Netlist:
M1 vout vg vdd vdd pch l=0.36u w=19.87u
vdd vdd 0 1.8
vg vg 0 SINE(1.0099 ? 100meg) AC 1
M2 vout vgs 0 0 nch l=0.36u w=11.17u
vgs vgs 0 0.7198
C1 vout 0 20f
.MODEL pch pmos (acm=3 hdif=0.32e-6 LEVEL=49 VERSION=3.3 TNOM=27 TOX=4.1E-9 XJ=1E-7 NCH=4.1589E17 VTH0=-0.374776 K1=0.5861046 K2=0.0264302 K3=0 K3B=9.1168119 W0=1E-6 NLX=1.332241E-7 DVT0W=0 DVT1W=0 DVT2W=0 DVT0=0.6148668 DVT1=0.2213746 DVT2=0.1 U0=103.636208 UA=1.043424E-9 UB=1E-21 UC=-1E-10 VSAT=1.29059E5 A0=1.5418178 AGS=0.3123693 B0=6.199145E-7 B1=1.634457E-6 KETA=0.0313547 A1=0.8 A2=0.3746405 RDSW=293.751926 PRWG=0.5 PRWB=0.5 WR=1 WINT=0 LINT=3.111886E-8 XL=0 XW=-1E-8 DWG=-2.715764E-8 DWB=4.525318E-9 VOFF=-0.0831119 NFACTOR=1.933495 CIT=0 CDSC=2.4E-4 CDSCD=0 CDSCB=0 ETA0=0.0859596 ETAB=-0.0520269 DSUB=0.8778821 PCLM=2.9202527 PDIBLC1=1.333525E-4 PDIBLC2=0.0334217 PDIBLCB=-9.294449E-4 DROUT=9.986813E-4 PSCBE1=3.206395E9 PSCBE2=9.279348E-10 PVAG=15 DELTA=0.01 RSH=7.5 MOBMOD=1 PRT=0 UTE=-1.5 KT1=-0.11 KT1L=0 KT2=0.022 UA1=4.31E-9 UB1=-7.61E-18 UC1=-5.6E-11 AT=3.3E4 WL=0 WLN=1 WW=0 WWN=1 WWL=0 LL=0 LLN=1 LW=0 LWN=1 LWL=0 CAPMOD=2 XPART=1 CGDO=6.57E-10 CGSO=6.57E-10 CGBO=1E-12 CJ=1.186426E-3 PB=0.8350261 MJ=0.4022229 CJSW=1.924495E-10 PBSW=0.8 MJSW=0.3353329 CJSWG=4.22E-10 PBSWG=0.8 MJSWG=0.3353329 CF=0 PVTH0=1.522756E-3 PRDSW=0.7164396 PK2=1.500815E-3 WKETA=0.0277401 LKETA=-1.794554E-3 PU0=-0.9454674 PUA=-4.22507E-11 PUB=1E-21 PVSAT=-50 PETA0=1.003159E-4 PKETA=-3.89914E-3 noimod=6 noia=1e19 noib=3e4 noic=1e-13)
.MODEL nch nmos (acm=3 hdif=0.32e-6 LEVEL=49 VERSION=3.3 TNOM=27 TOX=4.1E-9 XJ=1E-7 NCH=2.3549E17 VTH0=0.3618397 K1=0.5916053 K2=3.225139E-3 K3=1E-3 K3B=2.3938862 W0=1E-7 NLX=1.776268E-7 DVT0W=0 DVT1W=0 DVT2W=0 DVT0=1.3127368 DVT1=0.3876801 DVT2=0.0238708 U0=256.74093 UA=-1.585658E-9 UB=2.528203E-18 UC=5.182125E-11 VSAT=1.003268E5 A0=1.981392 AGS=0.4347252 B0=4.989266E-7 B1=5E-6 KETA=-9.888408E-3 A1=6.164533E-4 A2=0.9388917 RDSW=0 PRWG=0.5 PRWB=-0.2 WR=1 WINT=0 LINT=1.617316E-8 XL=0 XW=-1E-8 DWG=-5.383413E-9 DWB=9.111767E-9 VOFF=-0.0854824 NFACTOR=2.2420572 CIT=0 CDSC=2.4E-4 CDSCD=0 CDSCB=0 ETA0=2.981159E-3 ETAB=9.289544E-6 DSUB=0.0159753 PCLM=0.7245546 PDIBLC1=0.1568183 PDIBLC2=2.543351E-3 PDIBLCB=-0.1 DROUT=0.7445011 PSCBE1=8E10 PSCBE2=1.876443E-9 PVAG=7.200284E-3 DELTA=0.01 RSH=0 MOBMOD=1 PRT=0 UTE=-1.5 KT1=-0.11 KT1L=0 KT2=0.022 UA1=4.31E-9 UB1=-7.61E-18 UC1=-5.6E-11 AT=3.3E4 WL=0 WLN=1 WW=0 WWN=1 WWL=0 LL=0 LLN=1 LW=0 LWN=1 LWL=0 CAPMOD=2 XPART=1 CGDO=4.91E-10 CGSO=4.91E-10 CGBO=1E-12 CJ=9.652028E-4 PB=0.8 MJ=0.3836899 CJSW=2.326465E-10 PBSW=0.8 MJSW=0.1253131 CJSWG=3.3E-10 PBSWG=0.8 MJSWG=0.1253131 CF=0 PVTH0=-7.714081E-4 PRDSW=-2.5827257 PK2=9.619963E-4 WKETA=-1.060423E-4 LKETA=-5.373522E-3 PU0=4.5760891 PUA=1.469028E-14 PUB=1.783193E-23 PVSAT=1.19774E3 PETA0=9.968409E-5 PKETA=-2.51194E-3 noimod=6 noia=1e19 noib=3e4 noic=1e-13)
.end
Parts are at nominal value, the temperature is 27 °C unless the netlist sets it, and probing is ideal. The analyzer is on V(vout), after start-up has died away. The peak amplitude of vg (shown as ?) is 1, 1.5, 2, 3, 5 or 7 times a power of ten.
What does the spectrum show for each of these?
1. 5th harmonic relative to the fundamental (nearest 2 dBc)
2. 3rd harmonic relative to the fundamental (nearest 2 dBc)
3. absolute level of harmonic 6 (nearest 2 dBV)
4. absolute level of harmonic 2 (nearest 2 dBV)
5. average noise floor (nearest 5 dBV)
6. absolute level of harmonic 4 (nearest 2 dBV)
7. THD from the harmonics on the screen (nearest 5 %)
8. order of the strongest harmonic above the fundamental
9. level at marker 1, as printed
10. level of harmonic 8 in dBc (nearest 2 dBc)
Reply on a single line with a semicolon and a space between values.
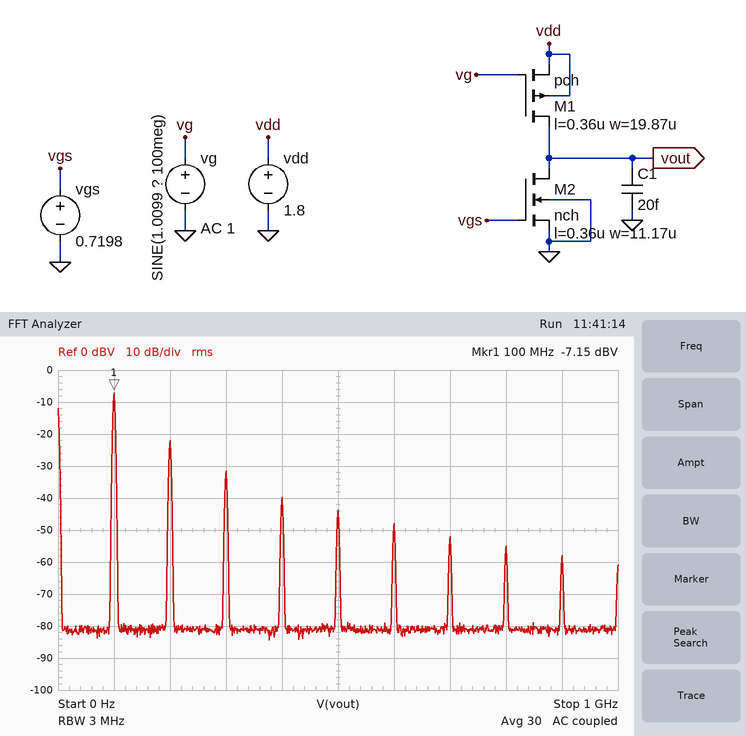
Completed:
-36 dBc; -24 dBc; -48 dBV; -22 dBV; -80 dBV; -40 dBV; 20 %; 2; -7.15 dBV; -48 dBc
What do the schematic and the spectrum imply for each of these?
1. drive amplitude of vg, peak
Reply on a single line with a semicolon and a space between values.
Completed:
50 mV
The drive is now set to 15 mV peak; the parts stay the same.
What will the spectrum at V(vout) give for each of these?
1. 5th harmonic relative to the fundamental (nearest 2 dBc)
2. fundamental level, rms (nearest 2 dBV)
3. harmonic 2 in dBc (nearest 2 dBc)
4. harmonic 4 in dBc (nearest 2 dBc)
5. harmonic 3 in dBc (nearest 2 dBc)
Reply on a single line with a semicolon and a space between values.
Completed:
-56 dBc; -16 dBV; -22 dBc; -46 dBc; -34 dBc
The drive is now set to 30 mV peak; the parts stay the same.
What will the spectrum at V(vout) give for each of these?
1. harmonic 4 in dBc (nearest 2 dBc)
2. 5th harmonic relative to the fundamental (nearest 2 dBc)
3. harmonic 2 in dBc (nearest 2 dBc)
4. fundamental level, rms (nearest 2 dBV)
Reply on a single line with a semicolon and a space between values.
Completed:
-36 dBc; -42 dBc; -16 dBc; -10 dBV
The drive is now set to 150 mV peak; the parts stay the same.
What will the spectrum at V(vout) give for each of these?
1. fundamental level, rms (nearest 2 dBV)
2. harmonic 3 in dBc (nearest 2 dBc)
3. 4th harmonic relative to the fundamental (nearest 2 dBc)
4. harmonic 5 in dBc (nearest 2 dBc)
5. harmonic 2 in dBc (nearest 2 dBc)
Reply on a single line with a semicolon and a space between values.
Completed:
-4 dBV; -14 dBc; -26 dBc; -24 dBc; -20 dBc
